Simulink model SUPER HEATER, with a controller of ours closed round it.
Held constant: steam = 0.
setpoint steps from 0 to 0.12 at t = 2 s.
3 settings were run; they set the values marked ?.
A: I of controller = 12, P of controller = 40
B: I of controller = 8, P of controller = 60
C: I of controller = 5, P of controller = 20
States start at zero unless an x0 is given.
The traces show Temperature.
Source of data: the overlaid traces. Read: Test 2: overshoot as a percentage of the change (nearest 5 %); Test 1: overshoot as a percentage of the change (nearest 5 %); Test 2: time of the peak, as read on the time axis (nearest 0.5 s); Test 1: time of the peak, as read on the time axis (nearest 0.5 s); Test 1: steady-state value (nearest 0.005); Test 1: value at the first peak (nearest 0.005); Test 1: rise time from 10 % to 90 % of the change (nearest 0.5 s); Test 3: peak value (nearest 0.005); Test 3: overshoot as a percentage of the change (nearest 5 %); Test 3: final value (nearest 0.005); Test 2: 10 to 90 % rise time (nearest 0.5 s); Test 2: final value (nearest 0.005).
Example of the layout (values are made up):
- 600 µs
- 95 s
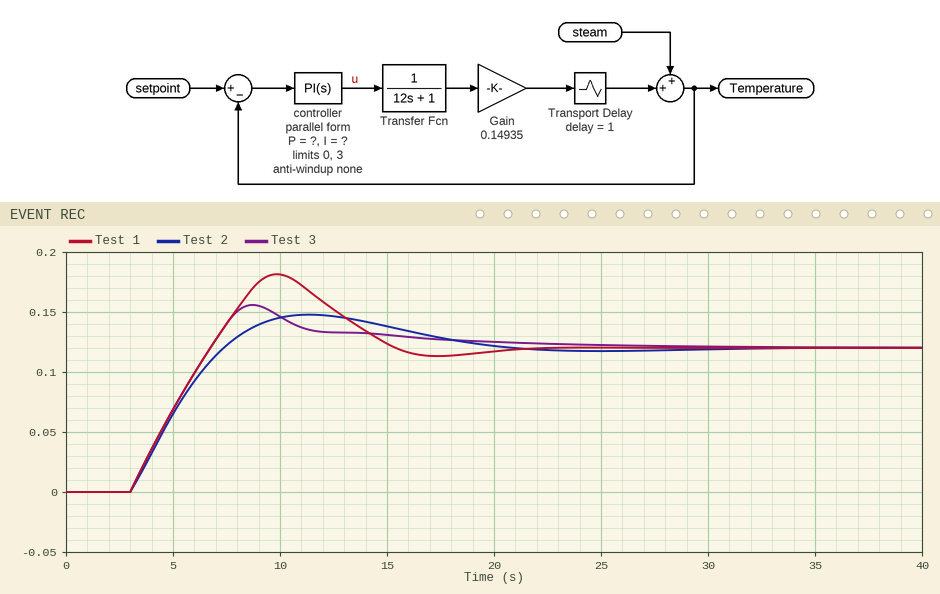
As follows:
- 25 %
- 50 %
- 11.5 s
- 10.0 s
- 0.120
- 0.180
- 3.0 s
- 0.155
- 30 %
- 0.120
- 3.5 s
- 0.120
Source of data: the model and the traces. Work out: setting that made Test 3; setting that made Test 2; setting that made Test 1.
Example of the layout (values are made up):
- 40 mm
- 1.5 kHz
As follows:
- B
- C
- A
